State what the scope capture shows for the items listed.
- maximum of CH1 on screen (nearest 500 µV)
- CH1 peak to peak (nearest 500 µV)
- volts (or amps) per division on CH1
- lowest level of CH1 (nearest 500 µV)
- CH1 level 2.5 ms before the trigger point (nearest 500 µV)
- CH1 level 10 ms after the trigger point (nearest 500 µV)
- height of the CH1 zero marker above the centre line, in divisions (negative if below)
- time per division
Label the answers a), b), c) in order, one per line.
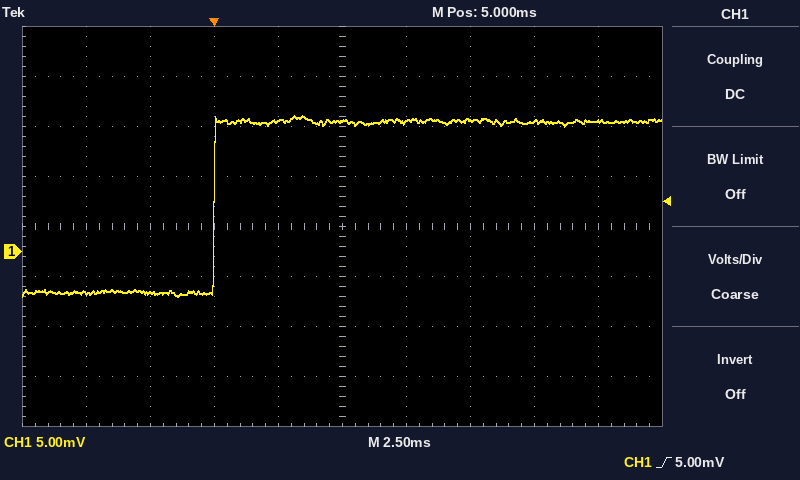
a) 13.5 mV
b) 18.0 mV
c) 5 mV
d) -4.5 mV
e) -4.0 mV
f) 13.0 mV
g) -0.5 div
h) 2.5 ms
